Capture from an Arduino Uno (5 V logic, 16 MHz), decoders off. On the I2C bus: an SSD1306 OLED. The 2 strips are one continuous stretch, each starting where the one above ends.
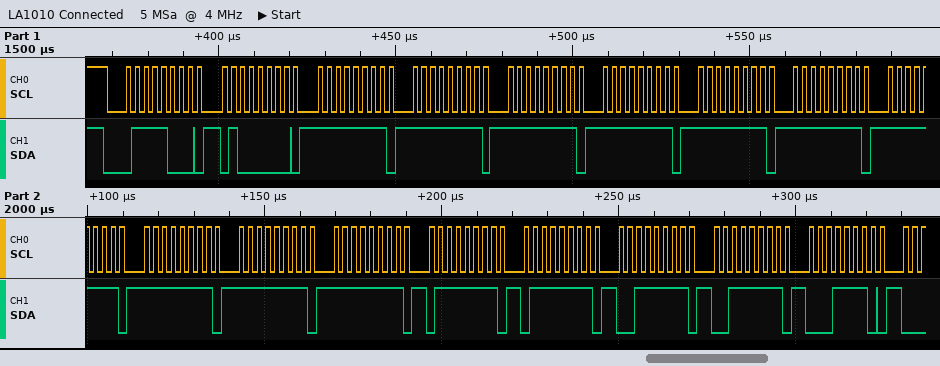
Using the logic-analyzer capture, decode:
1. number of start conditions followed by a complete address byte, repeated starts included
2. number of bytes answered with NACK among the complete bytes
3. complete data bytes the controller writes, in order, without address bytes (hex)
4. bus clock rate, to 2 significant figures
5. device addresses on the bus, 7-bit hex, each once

1
0
40 FF FF FF FF FF FF FF FF FF FF 7F 7F 3F 3F 1E
400 kHz
0x3C
